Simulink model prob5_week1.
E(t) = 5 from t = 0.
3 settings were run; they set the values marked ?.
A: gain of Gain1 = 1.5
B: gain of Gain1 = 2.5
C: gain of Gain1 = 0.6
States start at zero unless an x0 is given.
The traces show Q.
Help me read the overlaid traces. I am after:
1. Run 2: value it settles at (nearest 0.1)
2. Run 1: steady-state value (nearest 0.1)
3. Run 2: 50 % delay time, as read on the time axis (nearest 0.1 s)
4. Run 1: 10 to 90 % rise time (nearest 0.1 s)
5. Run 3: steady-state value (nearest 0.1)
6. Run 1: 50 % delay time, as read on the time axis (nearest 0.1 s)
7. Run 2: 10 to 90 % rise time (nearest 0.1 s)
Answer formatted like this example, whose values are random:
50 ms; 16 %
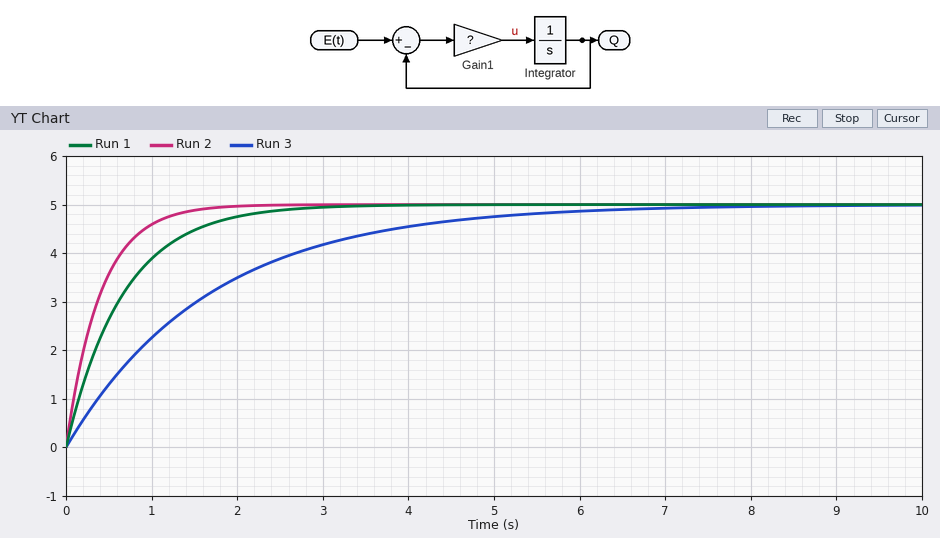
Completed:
5.0; 5.0; 0.3 s; 1.5 s; 5.0; 0.5 s; 0.9 s
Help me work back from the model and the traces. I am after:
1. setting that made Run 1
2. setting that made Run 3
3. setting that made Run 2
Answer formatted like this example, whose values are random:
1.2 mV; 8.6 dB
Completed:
A; C; B
